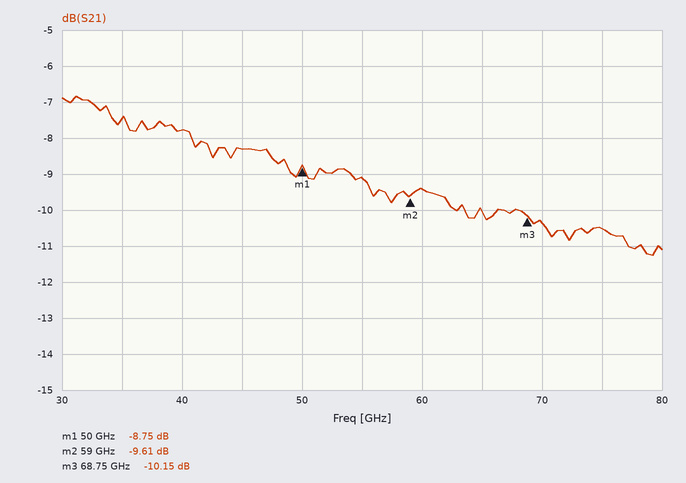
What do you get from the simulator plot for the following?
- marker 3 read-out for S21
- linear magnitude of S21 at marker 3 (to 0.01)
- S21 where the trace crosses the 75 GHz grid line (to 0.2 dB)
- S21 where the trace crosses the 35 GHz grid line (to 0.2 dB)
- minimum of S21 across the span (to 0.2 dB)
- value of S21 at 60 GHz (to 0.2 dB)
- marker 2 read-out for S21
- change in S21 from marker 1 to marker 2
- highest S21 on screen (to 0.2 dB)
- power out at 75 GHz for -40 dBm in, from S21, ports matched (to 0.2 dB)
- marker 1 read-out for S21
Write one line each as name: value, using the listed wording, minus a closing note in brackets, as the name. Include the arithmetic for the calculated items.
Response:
marker 3 read-out for S21: -10.15 dB
linear magnitude of S21 at marker 3: 10^(-10.15/20) ≈ 0.31
S21 where the trace crosses the 75 GHz grid line: -10.6 dB
S21 where the trace crosses the 35 GHz grid line: -7.4 dB
minimum of S21 across the span: -11.2 dB
value of S21 at 60 GHz: -9.4 dB
marker 2 read-out for S21: -9.61 dB
change in S21 from marker 1 to marker 2: -9.61 − (-8.75) = -0.86 dB
highest S21 on screen: -6.8 dB
power out at 75 GHz for -40 dBm in, from S21, ports matched: -40 dBm + (-10.6 dB) = -50.6 dBm
marker 1 read-out for S21: -8.75 dB
